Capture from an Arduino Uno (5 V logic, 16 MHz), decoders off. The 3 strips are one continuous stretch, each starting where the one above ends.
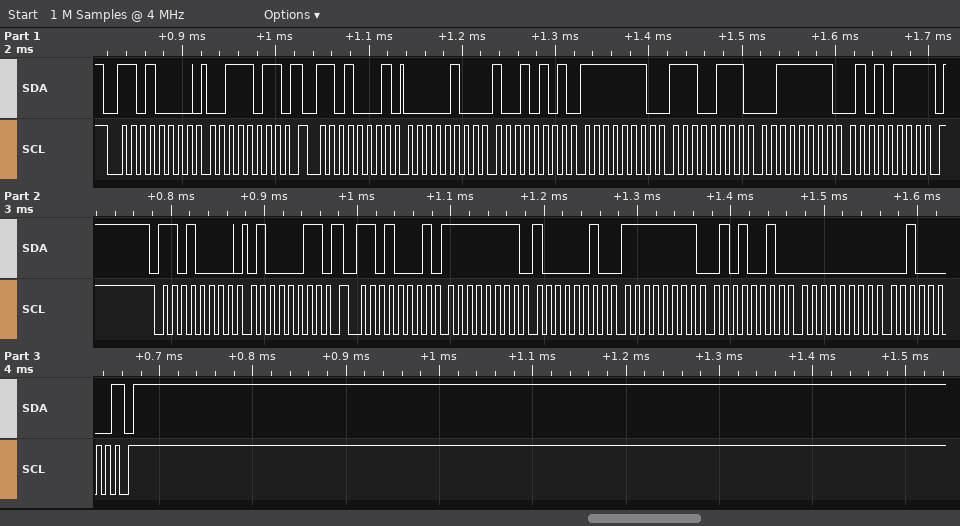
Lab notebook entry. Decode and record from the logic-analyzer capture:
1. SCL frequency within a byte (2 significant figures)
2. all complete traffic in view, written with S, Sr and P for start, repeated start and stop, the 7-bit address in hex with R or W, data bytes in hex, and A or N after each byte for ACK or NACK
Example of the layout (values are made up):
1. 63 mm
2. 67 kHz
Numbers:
1. 100 kHz
2. S 68W A 3B A Sr 68R A 04 A 95 A FE A E7 A 3F A 57 N P S 68W A 43 A Sr 68R A FF A 82 A FF A 52 A 00 A 20 N P
